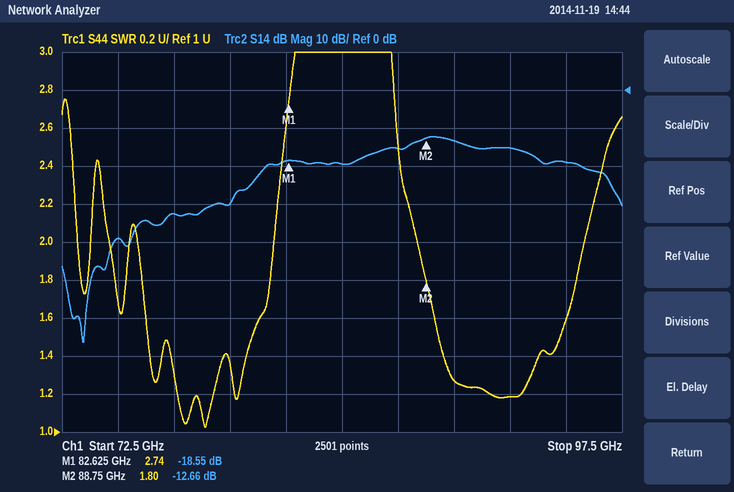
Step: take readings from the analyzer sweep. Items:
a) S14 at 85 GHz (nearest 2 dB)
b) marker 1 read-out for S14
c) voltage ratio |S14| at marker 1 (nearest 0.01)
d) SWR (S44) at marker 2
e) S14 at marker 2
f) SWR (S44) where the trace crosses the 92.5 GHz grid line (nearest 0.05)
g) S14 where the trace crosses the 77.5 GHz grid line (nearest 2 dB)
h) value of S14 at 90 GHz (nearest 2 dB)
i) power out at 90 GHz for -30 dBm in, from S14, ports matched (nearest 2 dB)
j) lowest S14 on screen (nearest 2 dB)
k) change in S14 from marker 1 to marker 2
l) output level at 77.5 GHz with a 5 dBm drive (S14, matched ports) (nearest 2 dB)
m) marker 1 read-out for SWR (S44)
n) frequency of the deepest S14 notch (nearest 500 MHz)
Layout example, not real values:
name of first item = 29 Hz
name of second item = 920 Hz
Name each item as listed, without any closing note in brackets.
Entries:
S14 at 85 GHz = -20 dB
marker 1 read-out for S14 = -18.55 dB
voltage ratio |S14| at marker 1 = 0.12
SWR (S44) at marker 2 = 1.80
S14 at marker 2 = -12.66 dB
SWR (S44) where the trace crosses the 92.5 GHz grid line = 1.20
S14 where the trace crosses the 77.5 GHz grid line = -32 dB
value of S14 at 90 GHz = -14 dB
power out at 90 GHz for -30 dBm in, from S14, ports matched = -44 dBm
lowest S14 on screen = -66 dB
change in S14 from marker 1 to marker 2 = 5.89 dB
output level at 77.5 GHz with a 5 dBm drive (S14, matched ports) = -28 dBm
marker 1 read-out for SWR = 2.74
frequency of the deepest S14 notch = 73.5 GHz
